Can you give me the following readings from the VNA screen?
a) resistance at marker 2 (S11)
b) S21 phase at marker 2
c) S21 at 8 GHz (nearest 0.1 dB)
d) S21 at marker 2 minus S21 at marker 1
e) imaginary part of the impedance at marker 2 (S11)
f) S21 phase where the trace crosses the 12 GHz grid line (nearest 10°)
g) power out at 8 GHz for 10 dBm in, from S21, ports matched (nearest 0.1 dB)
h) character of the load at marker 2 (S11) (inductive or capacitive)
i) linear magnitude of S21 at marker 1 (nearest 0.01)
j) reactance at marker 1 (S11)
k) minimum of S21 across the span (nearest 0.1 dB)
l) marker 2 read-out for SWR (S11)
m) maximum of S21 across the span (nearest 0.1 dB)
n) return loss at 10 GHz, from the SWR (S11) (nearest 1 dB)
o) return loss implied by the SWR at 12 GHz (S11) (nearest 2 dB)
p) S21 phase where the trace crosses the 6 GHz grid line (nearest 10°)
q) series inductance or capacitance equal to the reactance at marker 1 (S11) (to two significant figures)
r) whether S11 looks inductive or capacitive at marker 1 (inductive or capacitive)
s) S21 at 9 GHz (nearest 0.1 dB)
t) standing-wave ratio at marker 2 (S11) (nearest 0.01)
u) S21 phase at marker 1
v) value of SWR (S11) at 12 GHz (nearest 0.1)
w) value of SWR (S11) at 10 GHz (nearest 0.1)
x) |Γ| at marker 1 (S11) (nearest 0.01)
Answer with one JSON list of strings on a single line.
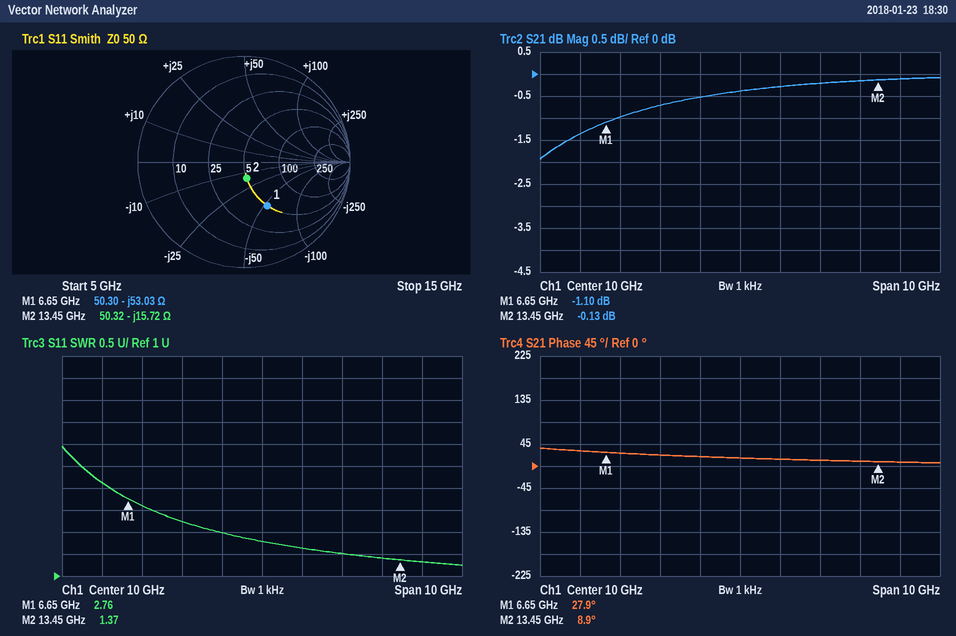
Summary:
["50.32 Ω", "8.9°", "-0.7 dB", "0.97 dB", "-15.72 Ω", "10°", "9.3 dBm", "capacitive", "0.88", "-53.03 Ω", "-1.9 dB", "1.37", "-0.1 dB", "11 dB", "14 dB", "30°", "450 fF", "capacitive", "-0.5 dB", "1.37", "27.9°", "1.5", "1.8", "0.47"]
